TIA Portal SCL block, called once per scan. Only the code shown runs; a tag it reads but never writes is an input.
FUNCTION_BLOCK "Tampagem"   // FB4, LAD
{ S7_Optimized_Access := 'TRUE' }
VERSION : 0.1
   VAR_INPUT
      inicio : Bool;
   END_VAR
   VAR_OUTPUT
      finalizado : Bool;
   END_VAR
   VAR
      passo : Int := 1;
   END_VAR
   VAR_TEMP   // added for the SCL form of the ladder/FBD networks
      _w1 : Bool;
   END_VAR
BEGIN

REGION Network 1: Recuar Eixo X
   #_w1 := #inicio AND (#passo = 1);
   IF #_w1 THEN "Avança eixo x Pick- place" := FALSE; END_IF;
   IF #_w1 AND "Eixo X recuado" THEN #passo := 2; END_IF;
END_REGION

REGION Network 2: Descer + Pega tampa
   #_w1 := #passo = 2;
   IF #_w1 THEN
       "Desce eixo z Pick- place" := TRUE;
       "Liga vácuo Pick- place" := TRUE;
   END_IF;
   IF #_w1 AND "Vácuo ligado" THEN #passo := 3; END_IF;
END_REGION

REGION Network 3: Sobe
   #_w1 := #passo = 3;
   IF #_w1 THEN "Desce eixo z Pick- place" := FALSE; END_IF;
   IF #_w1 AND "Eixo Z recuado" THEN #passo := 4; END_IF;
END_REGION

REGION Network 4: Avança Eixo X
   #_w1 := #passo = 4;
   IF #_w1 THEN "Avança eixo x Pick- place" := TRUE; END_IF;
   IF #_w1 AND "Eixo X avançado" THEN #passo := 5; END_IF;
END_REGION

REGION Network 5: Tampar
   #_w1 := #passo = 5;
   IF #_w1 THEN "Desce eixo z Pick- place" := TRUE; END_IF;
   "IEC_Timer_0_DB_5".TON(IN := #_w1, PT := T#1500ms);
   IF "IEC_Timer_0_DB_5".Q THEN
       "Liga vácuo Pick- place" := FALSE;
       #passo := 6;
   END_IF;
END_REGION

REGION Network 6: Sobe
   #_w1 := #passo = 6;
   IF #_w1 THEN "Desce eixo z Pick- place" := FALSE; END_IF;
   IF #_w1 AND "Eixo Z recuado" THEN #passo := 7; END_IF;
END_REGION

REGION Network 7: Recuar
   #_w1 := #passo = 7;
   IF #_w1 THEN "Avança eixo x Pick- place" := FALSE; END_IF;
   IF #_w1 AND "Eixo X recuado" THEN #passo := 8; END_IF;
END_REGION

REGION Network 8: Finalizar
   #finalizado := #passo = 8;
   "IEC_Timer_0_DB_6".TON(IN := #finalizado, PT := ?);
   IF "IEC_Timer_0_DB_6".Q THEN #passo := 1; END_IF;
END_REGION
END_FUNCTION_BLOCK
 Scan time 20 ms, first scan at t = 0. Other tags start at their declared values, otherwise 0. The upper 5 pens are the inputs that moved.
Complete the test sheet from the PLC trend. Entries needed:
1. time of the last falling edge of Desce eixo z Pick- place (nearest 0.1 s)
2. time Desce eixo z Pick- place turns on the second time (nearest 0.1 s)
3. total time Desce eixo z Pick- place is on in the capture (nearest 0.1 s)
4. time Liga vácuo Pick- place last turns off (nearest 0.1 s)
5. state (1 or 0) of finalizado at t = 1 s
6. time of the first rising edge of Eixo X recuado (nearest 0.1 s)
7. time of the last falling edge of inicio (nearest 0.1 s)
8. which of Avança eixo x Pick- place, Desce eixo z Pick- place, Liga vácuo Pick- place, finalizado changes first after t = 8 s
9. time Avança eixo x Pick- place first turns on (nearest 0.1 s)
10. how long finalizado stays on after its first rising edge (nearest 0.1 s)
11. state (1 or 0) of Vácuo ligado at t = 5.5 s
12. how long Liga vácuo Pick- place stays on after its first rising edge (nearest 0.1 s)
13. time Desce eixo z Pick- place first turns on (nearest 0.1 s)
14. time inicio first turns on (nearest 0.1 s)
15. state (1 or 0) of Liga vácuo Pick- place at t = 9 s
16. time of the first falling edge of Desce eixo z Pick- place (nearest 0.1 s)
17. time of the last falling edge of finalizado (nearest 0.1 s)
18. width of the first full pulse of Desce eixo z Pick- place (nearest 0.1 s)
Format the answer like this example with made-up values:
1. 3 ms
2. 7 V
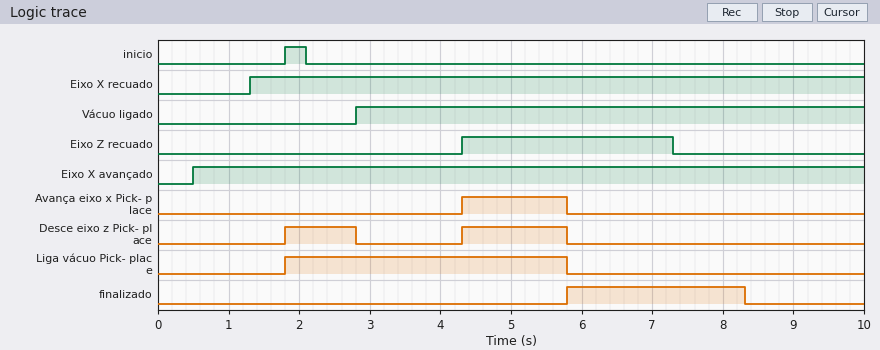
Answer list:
1. 5.8 s
2. 4.3 s
3. 2.5 s
4. 5.8 s
5. 0
6. 1.3 s
7. 2.1 s
8. finalizado
9. 4.3 s
10. 2.5 s
11. 1
12. 4.0 s
13. 1.8 s
14. 1.8 s
15. 0
16. 2.8 s
17. 8.3 s
18. 1.0 s
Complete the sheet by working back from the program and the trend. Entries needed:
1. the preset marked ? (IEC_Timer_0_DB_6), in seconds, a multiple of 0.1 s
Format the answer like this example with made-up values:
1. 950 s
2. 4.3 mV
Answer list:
1. 2.5 s
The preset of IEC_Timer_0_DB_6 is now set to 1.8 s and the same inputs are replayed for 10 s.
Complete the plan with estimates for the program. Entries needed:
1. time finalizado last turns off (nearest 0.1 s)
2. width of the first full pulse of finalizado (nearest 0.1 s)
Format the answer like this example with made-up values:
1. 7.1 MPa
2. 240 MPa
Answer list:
1. 7.6 s
2. 1.8 s
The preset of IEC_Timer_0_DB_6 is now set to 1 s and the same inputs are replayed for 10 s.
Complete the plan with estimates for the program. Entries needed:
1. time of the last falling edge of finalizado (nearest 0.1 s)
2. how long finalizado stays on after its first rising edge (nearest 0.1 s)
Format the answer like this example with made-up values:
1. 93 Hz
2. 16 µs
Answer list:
1. 6.8 s
2. 1.0 s
